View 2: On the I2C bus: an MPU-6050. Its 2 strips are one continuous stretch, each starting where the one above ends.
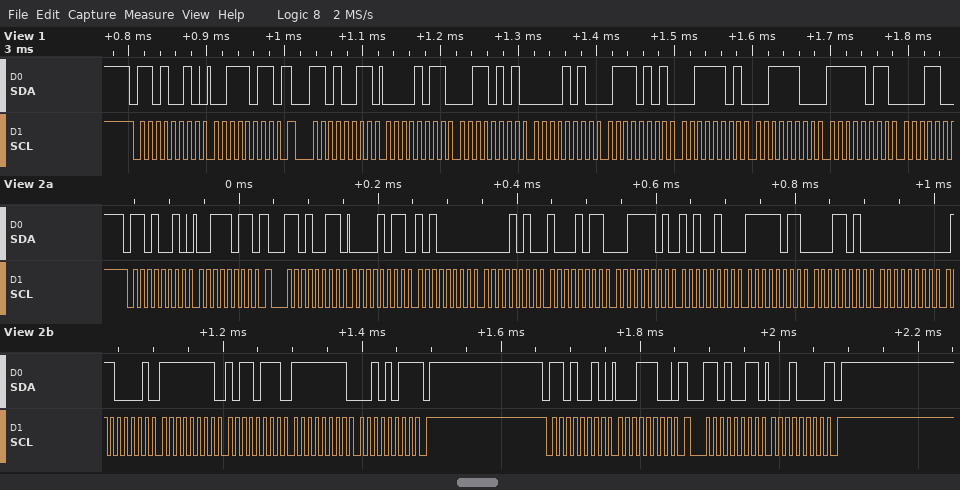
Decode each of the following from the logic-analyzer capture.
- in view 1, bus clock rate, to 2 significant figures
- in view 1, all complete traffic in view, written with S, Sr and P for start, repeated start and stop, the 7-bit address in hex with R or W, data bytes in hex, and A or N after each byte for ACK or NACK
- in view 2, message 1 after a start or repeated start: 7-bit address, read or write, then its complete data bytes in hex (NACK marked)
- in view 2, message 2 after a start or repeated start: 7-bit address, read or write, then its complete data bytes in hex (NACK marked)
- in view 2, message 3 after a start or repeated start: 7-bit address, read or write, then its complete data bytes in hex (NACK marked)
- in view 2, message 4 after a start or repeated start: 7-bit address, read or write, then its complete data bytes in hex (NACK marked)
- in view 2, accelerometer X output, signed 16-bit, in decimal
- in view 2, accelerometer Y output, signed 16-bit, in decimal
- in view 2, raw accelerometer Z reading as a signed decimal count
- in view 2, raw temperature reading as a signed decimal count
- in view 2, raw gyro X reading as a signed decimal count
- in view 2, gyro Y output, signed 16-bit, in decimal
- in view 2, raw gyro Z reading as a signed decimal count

100 kHz
S 69W A 3B A Sr 69R A 0B A 35 A 0A A 75 A 3D A 3C A FB A
0x69 write: 3B
0x69 read: 0B A0 0A 8B 3D A4 FB 1A 00 61 FF B7 FF 2B NACK
0x69 write: 1C
0x69 read: 10 NACK
2976
2699
15780
-1254
97
-73
-213
